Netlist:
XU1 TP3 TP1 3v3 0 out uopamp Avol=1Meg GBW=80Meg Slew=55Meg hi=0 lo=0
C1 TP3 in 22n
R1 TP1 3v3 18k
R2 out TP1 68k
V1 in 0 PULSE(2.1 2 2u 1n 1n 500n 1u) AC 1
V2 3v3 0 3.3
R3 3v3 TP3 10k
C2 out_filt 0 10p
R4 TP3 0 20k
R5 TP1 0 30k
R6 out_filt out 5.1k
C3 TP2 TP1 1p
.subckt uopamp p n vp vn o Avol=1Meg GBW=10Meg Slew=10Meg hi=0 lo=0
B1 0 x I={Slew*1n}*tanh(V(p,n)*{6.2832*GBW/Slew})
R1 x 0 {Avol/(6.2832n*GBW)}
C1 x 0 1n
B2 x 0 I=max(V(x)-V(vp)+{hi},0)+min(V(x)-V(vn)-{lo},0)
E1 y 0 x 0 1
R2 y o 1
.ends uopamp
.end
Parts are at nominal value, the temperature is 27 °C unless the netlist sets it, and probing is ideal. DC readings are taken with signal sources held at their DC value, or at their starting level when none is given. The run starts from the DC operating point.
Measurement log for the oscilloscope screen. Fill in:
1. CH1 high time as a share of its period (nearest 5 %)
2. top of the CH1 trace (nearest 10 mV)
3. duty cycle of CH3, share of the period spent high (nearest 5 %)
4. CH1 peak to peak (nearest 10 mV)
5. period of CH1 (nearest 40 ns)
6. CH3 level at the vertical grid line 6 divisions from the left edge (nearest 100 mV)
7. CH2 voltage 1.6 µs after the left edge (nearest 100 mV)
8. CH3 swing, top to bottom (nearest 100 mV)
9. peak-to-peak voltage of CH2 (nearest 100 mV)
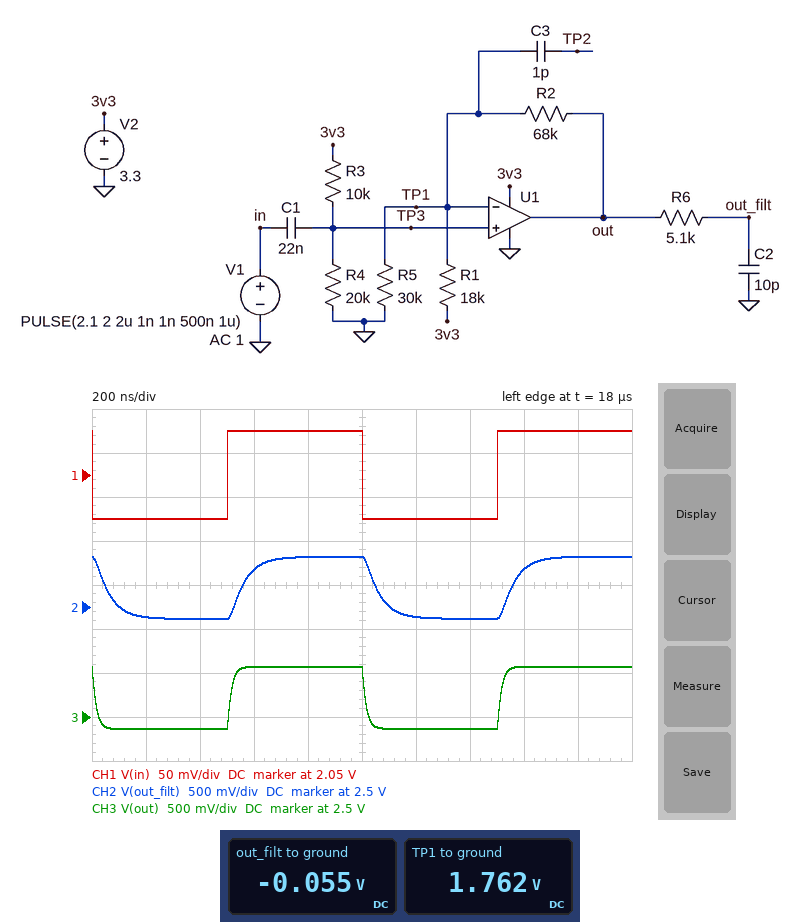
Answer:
50 %
2.10 V
50 %
100 mV
1.00 µs
2.4 V
2.9 V
700 mV
700 mV
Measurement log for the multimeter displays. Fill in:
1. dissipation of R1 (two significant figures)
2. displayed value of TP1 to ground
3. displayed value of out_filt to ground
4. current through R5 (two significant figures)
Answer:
130 µW
1.762 V
-0.055 V
59 µA
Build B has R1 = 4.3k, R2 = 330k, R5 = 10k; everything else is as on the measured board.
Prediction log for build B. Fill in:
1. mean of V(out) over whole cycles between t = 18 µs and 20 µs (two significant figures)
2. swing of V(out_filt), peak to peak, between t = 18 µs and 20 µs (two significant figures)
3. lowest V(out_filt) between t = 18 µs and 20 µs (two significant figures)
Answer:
-43 mV
17 mV
-51 mV
